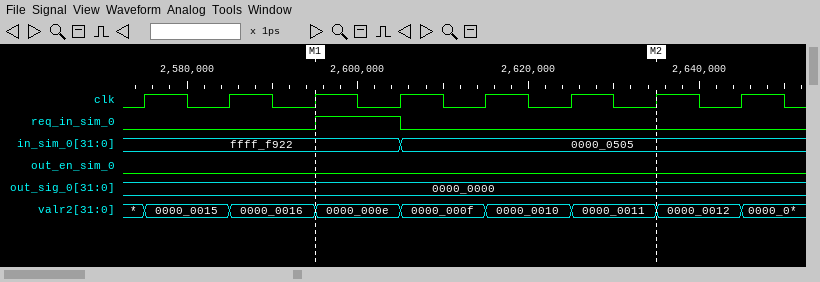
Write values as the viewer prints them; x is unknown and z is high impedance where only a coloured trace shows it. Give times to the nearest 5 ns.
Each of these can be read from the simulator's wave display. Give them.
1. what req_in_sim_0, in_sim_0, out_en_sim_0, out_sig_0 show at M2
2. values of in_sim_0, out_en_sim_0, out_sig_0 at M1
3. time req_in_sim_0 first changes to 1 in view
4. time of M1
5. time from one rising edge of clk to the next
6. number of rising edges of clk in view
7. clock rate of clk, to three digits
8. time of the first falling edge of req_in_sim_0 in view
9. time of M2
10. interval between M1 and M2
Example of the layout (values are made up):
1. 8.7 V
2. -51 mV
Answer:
1. req_in_sim_0=0, in_sim_0=0000_0505, out_en_sim_0=0, out_sig_0=0000_0000
2. in_sim_0=ffff_f922, out_en_sim_0=0, out_sig_0=0000_0000
3. 2595 ns
4. 2595 ns
5. 10 ns
6. 8
7. 100 MHz
8. 2605 ns
9. 2635 ns
10. 40 ns
